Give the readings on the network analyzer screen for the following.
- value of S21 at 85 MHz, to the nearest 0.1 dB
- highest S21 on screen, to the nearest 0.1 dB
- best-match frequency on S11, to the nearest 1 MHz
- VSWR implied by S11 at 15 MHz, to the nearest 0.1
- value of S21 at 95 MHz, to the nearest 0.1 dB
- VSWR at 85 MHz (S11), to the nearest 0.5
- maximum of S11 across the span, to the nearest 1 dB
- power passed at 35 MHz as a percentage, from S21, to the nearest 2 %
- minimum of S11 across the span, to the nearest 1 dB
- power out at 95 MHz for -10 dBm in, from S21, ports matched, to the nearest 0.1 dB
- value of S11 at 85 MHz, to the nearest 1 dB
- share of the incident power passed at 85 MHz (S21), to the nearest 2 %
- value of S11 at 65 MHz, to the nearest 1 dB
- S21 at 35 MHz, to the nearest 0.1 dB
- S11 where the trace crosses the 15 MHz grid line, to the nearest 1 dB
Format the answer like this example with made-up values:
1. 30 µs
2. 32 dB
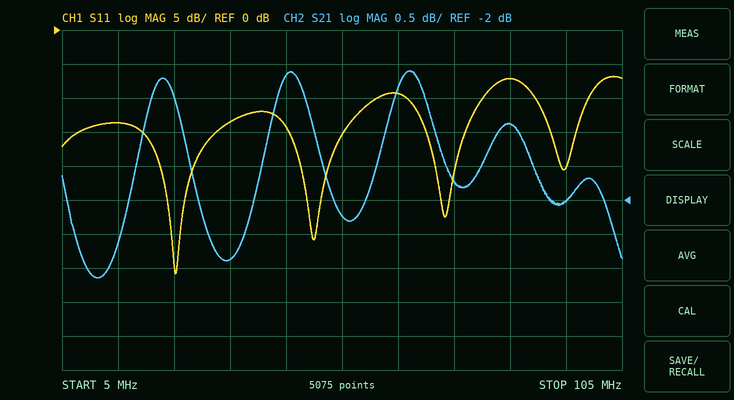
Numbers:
1. -0.9 dB
2. -0.1 dB
3. 25 MHz
4. 1.5
5. -2.0 dB
6. 2.5
7. -7 dB
8. 52 %
9. -36 dB
10. -12.0 dBm
11. -7 dB
12. 82 %
13. -9 dB
14. -2.9 dB
15. -14 dB
